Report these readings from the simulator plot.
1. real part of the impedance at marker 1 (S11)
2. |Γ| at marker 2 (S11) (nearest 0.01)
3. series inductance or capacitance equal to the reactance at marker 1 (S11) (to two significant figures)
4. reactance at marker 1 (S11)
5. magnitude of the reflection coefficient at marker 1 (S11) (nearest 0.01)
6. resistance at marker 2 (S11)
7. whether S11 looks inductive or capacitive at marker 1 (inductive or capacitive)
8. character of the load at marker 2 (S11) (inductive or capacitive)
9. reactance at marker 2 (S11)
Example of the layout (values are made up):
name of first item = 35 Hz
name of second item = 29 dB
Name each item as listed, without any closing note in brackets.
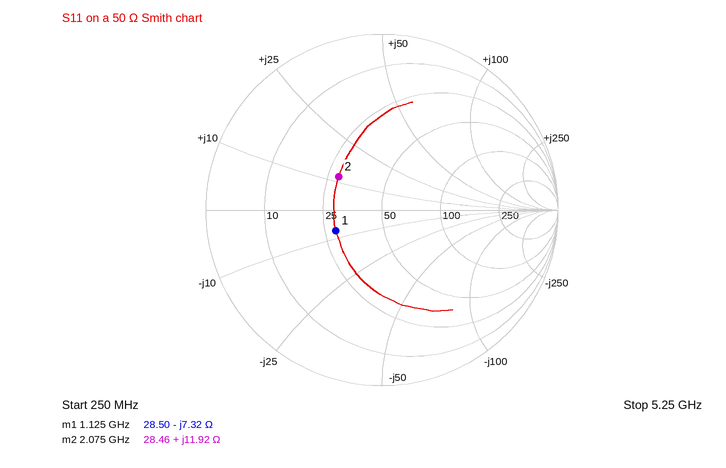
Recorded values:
real part of the impedance at marker 1 = 28.50 Ω
|Γ| at marker 2 (S11) = 0.31
series inductance or capacitance equal to the reactance at marker 1 (S11) = 19 pF
reactance at marker 1 = -7.32 Ω
magnitude of the reflection coefficient at marker 1 (S11) = 0.29
resistance at marker 2 = 28.46 Ω
whether S11 looks inductive or capacitive at marker 1 = capacitive
character of the load at marker 2 (S11) = inductive
reactance at marker 2 = +11.92 Ω
